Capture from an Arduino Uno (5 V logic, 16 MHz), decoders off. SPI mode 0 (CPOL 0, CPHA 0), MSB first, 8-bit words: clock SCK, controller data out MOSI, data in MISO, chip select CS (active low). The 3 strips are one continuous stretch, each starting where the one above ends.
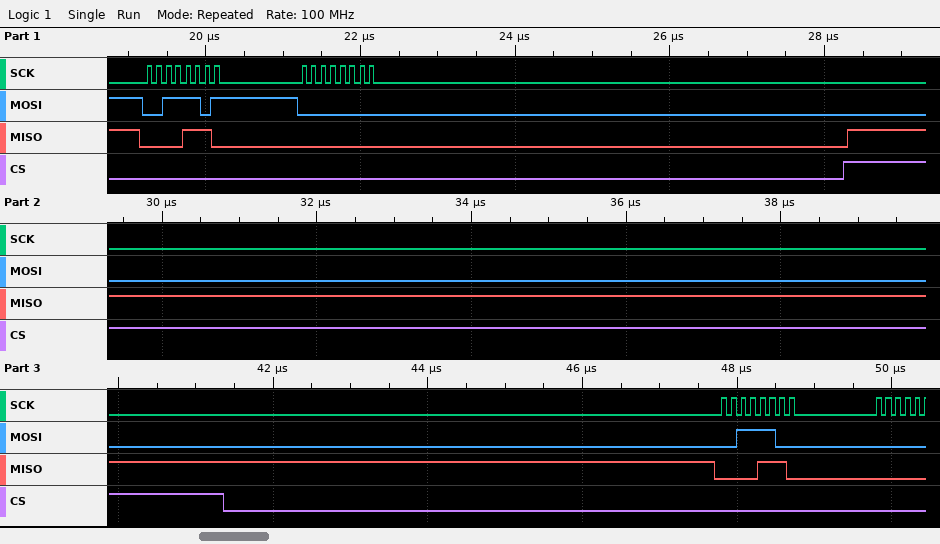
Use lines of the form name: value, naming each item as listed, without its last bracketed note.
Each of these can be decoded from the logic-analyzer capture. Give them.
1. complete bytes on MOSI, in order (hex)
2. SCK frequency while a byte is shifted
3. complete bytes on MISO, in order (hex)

complete bytes on MOSI, in order: 0x3D 0x00 0x3C
SCK frequency while a byte is shifted: 8 MHz
complete bytes on MISO, in order: 0x0E 0x00 0x0E
